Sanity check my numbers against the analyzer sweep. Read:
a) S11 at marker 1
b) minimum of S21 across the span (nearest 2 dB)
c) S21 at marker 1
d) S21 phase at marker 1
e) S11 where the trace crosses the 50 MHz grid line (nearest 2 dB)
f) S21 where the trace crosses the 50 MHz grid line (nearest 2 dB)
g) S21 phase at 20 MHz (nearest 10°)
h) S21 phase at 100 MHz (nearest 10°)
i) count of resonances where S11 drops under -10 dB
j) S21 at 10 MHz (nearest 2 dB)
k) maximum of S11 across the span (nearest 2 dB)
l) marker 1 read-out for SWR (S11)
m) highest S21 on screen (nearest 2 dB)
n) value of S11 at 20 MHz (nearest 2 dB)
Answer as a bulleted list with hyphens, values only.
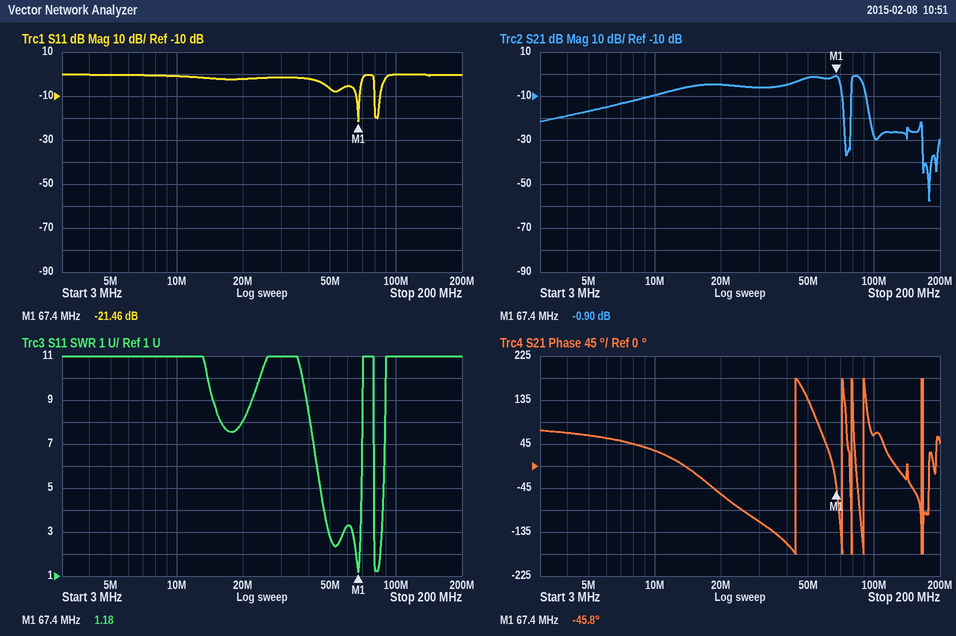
- -21.46 dB
- -58 dB
- -0.90 dB
- -45.8°
- -6 dB
- -2 dB
- -60°
- 60°
- 2
- -10 dB
- 0 dB
- 1.18
- 0 dB
- -2 dB
